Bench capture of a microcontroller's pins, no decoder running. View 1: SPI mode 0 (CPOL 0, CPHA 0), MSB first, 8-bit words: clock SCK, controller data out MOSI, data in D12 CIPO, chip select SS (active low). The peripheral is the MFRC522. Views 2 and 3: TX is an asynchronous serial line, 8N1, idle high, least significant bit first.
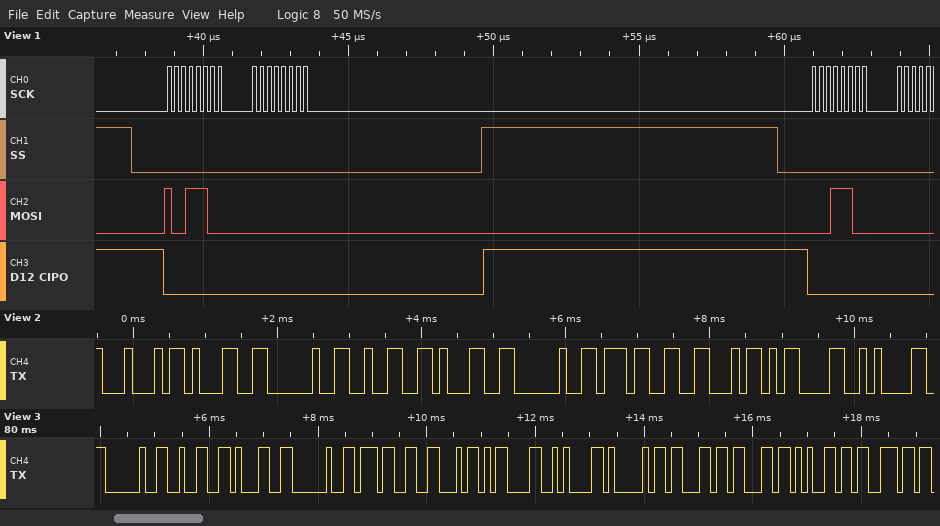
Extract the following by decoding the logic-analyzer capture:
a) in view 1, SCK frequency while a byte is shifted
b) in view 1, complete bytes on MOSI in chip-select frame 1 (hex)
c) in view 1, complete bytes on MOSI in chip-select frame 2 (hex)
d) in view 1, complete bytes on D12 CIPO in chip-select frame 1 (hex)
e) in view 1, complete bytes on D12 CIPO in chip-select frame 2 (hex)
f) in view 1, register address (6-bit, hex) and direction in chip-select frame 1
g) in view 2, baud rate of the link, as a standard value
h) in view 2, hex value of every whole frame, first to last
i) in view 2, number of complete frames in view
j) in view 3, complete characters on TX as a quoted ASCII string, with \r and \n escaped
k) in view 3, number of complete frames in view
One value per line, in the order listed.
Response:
4 MHz
9C 00
1C
00 00
00
0x0E read
9600 baud
44 31 20 32 31 20 37 46 0D 0A
10
" 21 7F\r\nAcces"
13
